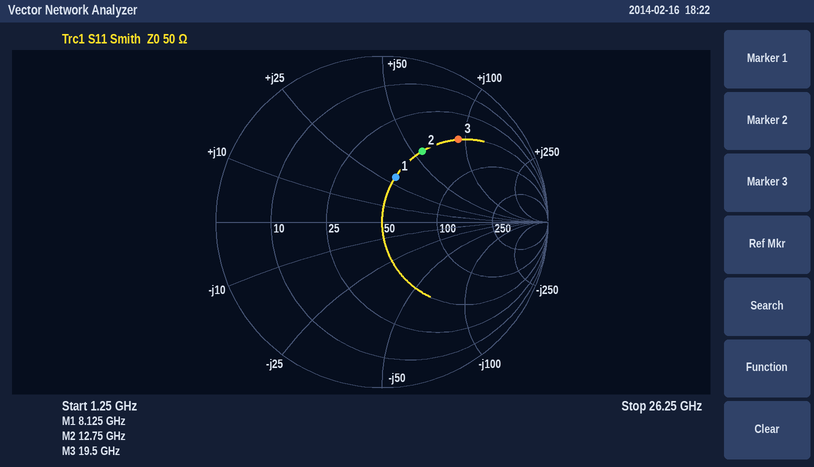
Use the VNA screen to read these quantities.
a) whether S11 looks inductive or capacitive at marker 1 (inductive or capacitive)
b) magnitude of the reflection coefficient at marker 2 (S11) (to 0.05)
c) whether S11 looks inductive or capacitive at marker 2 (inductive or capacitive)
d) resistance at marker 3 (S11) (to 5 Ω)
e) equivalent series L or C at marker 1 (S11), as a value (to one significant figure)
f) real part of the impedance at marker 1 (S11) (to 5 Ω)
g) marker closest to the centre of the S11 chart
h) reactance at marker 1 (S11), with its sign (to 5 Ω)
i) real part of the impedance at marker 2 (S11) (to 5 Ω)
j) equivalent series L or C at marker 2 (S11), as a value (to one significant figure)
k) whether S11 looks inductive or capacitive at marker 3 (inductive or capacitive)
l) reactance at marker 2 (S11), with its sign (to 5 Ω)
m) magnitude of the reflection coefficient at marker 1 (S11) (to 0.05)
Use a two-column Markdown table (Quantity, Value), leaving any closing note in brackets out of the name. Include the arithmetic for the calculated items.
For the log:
| Quantity | Value |
|---|---|
| whether S11 looks inductive or capacitive at marker 1 | inductive |
| magnitude of the reflection coefficient at marker 2 (S11) | 0.50 |
| whether S11 looks inductive or capacitive at marker 2 | inductive |
| resistance at marker 3 (S11) | 50 Ω |
| equivalent series L or C at marker 1 (S11), as a value | L = 30 Ω/(2π × 8.125 GHz) ≈ 588 pH, so 600 pH to one significant figure |
| real part of the impedance at marker 1 (S11) | 50 Ω |
| marker closest to the centre of the S11 chart | marker 1 |
| reactance at marker 1 (S11), with its sign | +30 Ω |
| real part of the impedance at marker 2 (S11) | 50 Ω |
| equivalent series L or C at marker 2 (S11), as a value | L = 55 Ω/(2π × 12.75 GHz) ≈ 687 pH, so 700 pH to one significant figure |
| whether S11 looks inductive or capacitive at marker 3 | inductive |
| reactance at marker 2 (S11), with its sign | +55 Ω |
| magnitude of the reflection coefficient at marker 1 (S11) | 0.30 |
